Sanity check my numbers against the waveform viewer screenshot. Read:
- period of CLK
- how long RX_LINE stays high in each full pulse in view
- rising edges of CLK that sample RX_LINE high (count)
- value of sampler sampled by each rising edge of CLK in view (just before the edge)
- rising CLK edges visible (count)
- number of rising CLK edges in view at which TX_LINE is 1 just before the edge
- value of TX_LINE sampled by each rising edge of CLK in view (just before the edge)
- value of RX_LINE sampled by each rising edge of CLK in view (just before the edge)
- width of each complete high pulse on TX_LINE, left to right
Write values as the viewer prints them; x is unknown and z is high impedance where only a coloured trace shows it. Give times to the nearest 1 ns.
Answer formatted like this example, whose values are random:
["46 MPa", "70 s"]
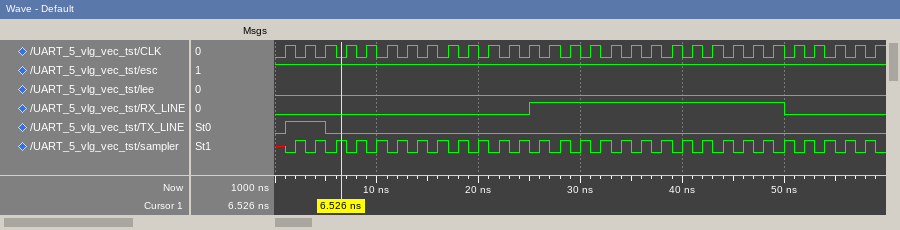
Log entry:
["2 ns", "25 ns", "12", "x 1 1 1 1 1 1 1 1 1 1 1 1 1 1 1 1 1 1 1 1 1 1 1 1 1 1 1 1 1", "30", "2", "0 1 1 0 0 0 0 0 0 0 0 0 0 0 0 0 0 0 0 0 0 0 0 0 0 0 0 0 0 0", "0 0 0 0 0 0 0 0 0 0 0 0 0 1 1 1 1 1 1 1 1 1 1 1 1 0 0 0 0 0", "4 ns"]
